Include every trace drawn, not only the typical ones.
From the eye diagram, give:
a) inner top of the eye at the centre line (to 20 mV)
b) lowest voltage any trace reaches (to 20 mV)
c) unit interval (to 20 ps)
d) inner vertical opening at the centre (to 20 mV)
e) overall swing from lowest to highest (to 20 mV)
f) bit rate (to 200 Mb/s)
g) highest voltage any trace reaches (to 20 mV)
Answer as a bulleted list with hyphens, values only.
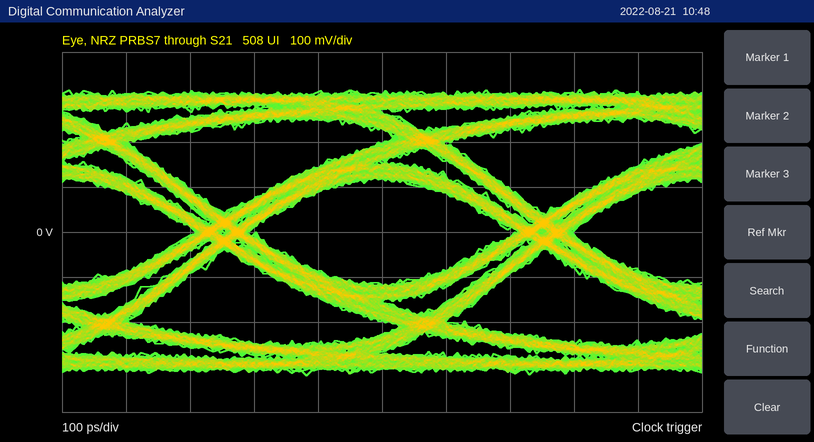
- 120 mV
- -320 mV
- 500 ps
- 240 mV
- 640 mV
- 2.0 Gb/s
- 320 mV
